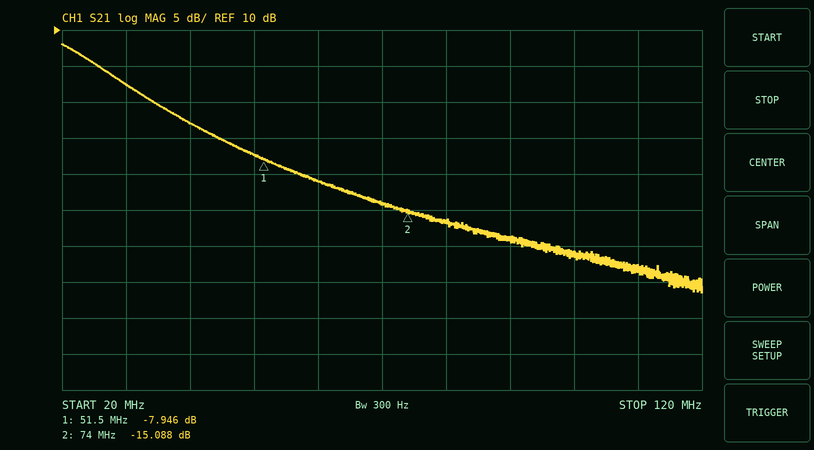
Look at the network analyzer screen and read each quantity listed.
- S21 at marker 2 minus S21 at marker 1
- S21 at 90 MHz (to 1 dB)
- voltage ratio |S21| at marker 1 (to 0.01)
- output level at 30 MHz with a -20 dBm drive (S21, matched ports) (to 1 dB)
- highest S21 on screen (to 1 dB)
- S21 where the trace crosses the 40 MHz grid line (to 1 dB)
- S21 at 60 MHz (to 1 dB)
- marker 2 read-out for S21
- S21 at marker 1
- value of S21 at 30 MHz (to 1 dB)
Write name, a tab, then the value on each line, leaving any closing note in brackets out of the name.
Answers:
S21 at marker 2 minus S21 at marker 1	-7.142 dB
S21 at 90 MHz	-19 dB
voltage ratio |S21| at marker 1	0.40
output level at 30 MHz with a -20 dBm drive (S21, matched ports)	-18 dBm
highest S21 on screen	8 dB
S21 where the trace crosses the 40 MHz grid line	-3 dB
S21 at 60 MHz	-11 dB
marker 2 read-out for S21	-15.088 dB
S21 at marker 1	-7.946 dB
value of S21 at 30 MHz	2 dB
